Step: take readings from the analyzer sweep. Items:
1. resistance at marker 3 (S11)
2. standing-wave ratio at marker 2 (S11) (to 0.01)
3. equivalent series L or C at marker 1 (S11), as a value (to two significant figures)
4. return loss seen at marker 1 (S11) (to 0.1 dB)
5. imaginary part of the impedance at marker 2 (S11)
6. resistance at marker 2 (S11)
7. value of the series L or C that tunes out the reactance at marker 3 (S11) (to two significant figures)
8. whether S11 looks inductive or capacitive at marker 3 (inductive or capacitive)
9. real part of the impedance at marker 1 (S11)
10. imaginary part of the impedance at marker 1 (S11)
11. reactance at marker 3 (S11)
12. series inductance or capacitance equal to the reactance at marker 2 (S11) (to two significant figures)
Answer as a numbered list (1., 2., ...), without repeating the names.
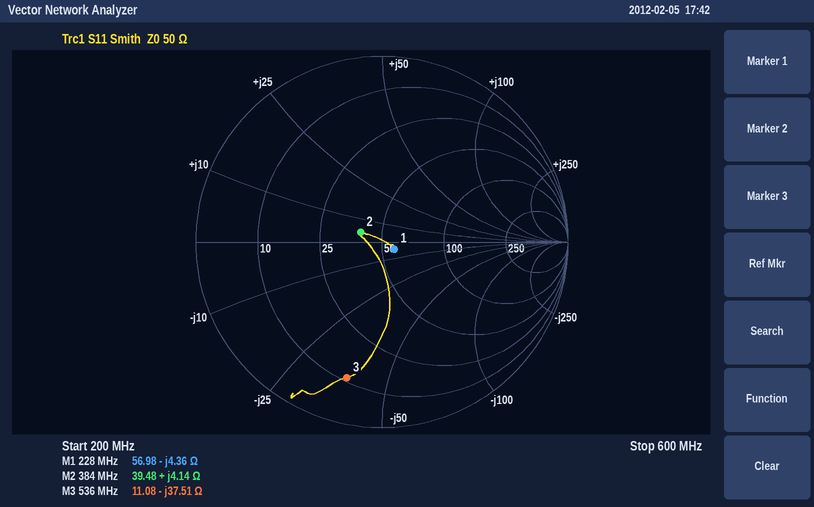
1. 11.08 Ω
2. 1.29
3. 160 pF
4. 22.3 dB
5. +4.14 Ω
6. 39.48 Ω
7. 11 nH
8. capacitive
9. 56.98 Ω
10. -4.36 Ω
11. -37.51 Ω
12. 1.7 nH
